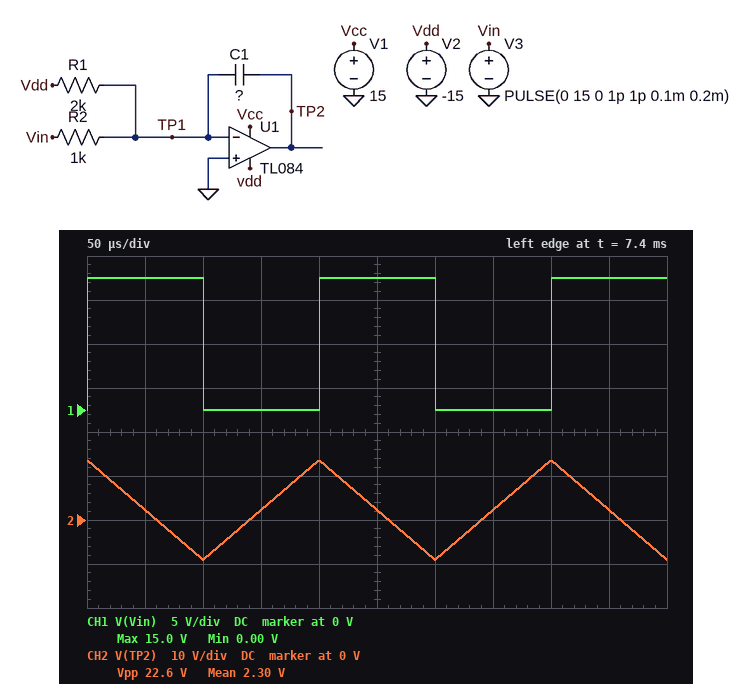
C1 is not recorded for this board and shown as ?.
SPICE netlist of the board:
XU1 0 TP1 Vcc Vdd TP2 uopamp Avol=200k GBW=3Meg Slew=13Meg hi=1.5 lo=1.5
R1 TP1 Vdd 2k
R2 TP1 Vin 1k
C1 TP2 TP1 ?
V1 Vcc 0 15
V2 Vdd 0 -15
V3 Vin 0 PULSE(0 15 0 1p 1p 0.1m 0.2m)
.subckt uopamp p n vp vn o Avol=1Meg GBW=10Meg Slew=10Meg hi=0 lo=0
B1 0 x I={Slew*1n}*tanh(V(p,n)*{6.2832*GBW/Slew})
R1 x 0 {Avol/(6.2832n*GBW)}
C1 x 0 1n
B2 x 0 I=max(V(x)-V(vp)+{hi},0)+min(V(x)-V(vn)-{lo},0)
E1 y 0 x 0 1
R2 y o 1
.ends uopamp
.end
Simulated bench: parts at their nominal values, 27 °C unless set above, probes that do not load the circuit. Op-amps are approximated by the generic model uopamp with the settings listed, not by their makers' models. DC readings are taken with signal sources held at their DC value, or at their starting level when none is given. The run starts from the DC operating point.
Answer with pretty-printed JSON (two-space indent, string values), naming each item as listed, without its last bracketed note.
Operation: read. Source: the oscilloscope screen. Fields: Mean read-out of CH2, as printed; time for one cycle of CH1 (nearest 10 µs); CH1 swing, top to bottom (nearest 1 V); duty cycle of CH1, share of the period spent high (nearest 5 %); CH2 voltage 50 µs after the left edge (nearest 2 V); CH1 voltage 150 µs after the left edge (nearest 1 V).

{
  "Mean read-out of CH2, as printed": "2.30 V",
  "time for one cycle of CH1": "200 µs",
  "CH1 swing, top to bottom": "15 V",
  "duty cycle of CH1, share of the period spent high": "50 %",
  "CH2 voltage 50 µs after the left edge": "2 V",
  "CH1 voltage 150 µs after the left edge": "0 V"
}
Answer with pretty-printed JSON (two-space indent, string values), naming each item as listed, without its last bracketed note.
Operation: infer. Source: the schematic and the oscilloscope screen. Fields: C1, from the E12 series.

{
  "C1, from the E12 series": "33 nF"
}
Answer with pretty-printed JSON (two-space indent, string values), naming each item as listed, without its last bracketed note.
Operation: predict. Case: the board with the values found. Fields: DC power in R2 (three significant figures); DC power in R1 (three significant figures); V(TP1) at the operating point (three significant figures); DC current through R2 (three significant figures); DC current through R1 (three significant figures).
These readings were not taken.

{
  "DC power in R2": "25.0 mW",
  "DC power in R1": "50.0 mW",
  "V(TP1) at the operating point": "-5.00 V",
  "DC current through R2": "5.00 mA",
  "DC current through R1": "5.00 mA"
}
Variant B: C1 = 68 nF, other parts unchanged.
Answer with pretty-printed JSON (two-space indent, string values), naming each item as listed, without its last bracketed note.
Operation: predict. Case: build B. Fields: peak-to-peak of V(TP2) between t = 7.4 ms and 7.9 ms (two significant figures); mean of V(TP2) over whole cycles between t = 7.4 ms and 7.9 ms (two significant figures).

{
  "peak-to-peak of V(TP2) between t = 7.4 ms and 7.9 ms": "11 V",
  "mean of V(TP2) over whole cycles between t = 7.4 ms and 7.9 ms": "8.1 V"
}
